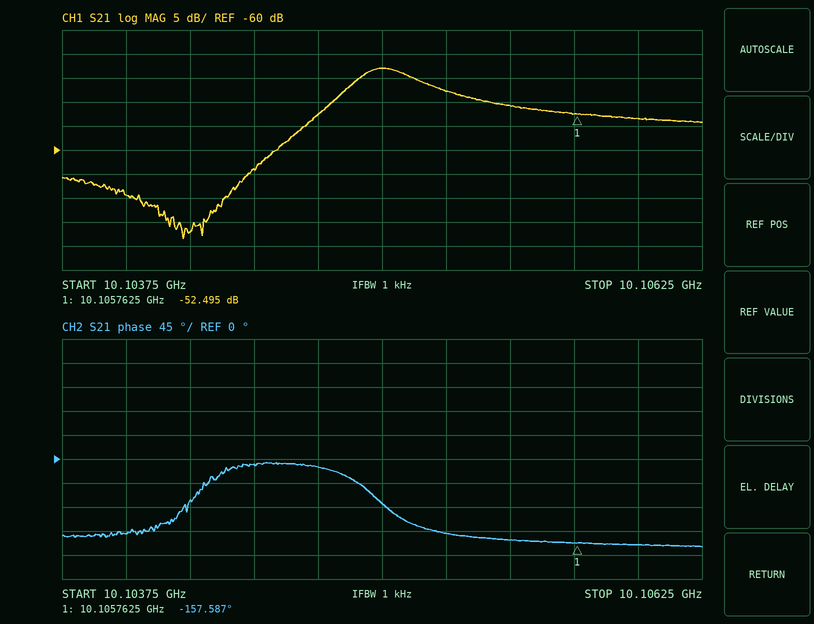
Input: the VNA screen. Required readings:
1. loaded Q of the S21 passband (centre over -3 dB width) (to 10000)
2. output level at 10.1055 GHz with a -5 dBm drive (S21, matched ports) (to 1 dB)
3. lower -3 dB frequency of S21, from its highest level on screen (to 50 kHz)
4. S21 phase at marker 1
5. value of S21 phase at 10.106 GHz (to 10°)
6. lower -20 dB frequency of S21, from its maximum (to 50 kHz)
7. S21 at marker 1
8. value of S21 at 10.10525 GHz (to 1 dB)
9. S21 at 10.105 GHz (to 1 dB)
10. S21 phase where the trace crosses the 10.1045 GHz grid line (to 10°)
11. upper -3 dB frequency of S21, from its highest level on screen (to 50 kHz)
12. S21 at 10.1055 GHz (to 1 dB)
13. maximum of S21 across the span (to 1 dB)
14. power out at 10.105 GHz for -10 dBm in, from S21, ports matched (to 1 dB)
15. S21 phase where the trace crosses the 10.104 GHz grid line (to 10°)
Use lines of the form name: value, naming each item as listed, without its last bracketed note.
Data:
loaded Q of the S21 passband (centre over -3 dB width): 40000
output level at 10.1055 GHz with a -5 dBm drive (S21, matched ports): -56 dBm
lower -3 dB frequency of S21, from its highest level on screen: 10.10490 GHz
S21 phase at marker 1: -157.587°
value of S21 phase at 10.106 GHz: -160°
lower -20 dB frequency of S21, from its maximum: 10.10450 GHz
S21 at marker 1: -52.495 dB
value of S21 at 10.10525 GHz: -48 dB
S21 at 10.105 GHz: -43 dB
S21 phase where the trace crosses the 10.1045 GHz grid line: -10°
upper -3 dB frequency of S21, from its highest level on screen: 10.10515 GHz
S21 at 10.1055 GHz: -51 dB
maximum of S21 across the span: -43 dB
power out at 10.105 GHz for -10 dBm in, from S21, ports matched: -53 dBm
S21 phase where the trace crosses the 10.104 GHz grid line: -140°
